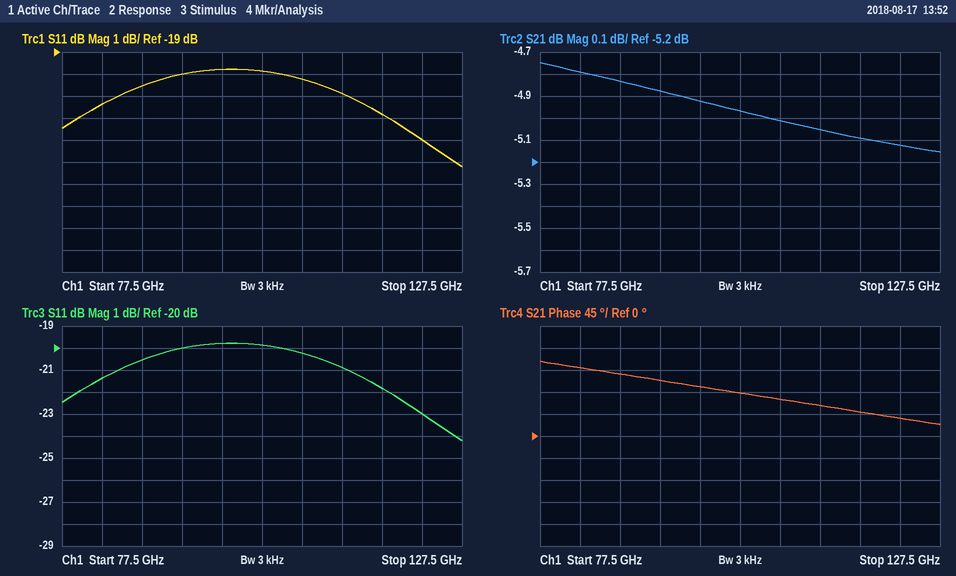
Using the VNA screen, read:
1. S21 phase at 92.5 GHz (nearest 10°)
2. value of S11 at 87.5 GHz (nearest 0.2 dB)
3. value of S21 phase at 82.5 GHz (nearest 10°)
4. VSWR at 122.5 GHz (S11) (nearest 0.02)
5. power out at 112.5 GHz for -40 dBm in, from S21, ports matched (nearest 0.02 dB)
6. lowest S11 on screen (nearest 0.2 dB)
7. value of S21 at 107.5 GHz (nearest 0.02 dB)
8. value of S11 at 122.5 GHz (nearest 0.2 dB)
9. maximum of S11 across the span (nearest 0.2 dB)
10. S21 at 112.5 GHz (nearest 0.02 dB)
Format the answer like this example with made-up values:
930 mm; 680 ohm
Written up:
110°; -20.6 dB; 140°; 1.16; -45.06 dBm; -24.2 dB; -5.02 dB; -23.0 dB; -19.8 dB; -5.06 dB
